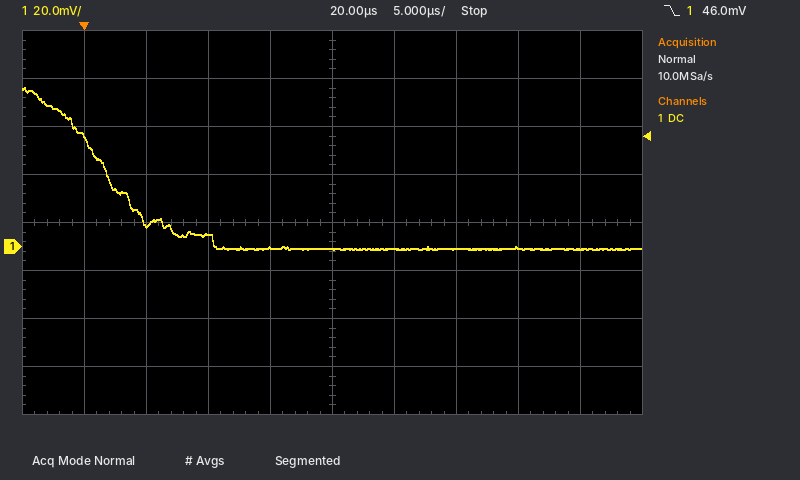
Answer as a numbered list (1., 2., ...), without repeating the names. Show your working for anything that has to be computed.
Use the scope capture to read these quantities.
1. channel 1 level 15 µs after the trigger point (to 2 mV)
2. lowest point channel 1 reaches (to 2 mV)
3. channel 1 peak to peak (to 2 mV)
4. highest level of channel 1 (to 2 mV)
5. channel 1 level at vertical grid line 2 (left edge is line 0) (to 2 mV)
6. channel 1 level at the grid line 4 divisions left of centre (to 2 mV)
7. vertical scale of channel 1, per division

1. 0 mV
2. -2 mV
3. 66 mV − (-2 mV) = 68 mV
4. 66 mV
5. 10 mV
6. 46 mV
7. 20 mV
